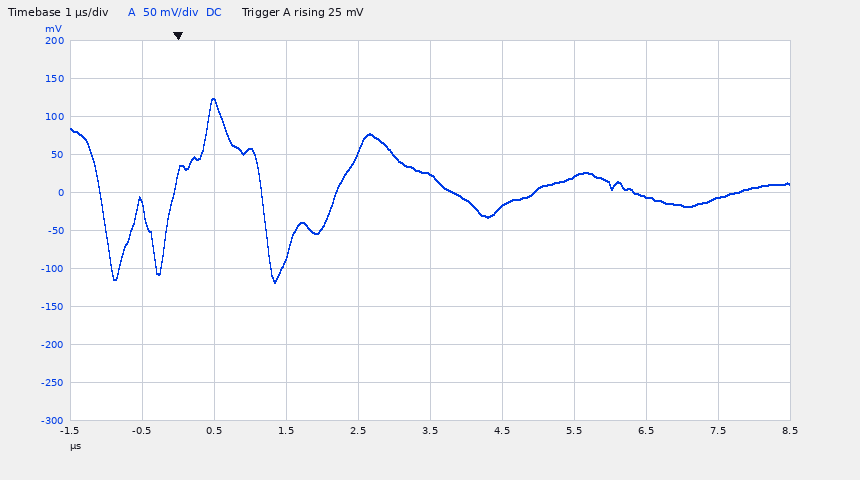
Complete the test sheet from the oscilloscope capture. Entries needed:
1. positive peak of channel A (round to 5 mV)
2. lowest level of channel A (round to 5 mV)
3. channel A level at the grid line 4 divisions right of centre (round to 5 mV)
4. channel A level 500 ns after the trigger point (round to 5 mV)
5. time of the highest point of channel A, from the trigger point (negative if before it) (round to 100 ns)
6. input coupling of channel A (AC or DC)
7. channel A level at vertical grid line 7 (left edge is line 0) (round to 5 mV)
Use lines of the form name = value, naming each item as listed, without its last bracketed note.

positive peak of channel A = 125 mV
lowest level of channel A = -120 mV
channel A level at the grid line 4 divisions right of centre = -5 mV
channel A level 500 ns after the trigger point = 120 mV
time of the highest point of channel A, from the trigger point (negative if before it) = +500 ns
input coupling of channel A = DC
channel A level at vertical grid line 7 (left edge is line 0) = 20 mV
